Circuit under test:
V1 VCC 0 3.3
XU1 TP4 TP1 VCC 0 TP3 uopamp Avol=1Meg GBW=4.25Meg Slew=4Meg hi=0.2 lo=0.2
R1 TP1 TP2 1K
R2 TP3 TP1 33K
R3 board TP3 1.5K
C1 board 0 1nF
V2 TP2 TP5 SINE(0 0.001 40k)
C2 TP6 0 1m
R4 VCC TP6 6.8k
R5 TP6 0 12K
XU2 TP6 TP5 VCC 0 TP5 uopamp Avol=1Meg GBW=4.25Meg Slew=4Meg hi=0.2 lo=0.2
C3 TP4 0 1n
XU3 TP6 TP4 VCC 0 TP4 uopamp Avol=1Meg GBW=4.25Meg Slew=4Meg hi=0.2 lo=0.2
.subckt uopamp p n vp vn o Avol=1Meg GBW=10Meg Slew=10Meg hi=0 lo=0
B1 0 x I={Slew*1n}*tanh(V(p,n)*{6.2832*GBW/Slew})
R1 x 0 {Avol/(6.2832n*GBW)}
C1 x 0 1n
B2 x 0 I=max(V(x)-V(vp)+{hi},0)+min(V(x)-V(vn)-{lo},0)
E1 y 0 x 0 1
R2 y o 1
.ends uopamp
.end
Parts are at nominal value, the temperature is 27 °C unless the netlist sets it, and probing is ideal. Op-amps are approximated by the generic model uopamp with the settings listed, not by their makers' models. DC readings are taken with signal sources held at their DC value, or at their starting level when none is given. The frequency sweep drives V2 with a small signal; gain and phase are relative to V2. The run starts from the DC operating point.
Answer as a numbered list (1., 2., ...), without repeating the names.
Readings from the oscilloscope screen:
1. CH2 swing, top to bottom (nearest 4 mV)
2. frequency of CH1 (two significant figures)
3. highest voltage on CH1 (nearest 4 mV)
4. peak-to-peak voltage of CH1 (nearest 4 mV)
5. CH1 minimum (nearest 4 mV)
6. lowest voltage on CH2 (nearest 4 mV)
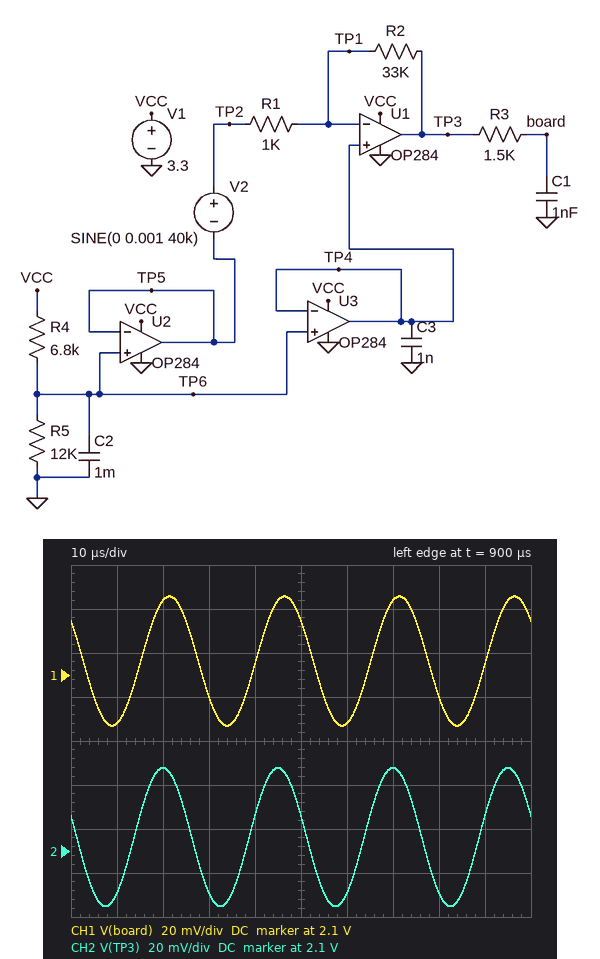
1. 64 mV
2. 40 kHz
3. 2.136 V
4. 60 mV
5. 2.076 V
6. 2.076 V
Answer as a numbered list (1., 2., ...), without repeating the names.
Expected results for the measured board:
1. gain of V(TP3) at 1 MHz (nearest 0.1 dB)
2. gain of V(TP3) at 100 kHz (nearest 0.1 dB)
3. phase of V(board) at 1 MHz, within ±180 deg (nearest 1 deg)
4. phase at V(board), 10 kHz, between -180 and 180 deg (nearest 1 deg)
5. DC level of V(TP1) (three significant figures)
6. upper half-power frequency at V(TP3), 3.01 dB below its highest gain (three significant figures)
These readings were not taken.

1. 12.2 dB
2. 28.2 dB
3. 13 deg
4. 170 deg
5. 2.11 V
6. 125 kHz
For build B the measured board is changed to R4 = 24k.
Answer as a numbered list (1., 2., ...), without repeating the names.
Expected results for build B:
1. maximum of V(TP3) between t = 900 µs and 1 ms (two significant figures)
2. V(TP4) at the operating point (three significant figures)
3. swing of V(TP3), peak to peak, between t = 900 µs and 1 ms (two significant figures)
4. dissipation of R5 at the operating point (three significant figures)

1. 1.1 V
2. 1.10 V
3. 63 mV
4. 101 µW
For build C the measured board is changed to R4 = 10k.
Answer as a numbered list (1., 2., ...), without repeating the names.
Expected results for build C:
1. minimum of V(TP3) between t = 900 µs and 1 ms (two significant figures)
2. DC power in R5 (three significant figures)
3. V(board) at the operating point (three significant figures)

1. 1.8 V
2. 270 µW
3. 1.80 V
